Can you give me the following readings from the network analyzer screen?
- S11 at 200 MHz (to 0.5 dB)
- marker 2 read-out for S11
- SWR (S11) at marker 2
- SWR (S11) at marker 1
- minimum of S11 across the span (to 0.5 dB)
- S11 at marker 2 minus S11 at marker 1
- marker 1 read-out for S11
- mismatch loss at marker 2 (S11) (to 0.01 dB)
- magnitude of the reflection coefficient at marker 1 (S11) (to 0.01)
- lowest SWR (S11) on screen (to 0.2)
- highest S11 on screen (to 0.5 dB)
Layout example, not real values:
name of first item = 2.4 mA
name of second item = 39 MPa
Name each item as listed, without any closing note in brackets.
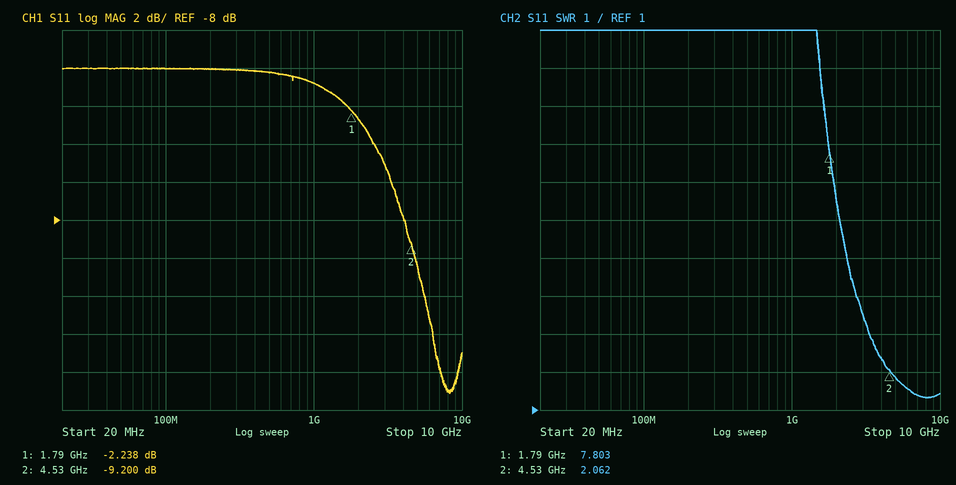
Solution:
S11 at 200 MHz = 0.0 dB
marker 2 read-out for S11 = -9.200 dB
SWR (S11) at marker 2 = 2.062
SWR (S11) at marker 1 = 7.803
minimum of S11 across the span = -17.0 dB
S11 at marker 2 minus S11 at marker 1 = -6.962 dB
marker 1 read-out for S11 = -2.238 dB
mismatch loss at marker 2 (S11) = 0.56 dB
magnitude of the reflection coefficient at marker 1 (S11) = 0.77
lowest SWR (S11) on screen = 1.4
highest S11 on screen = 0.0 dB
